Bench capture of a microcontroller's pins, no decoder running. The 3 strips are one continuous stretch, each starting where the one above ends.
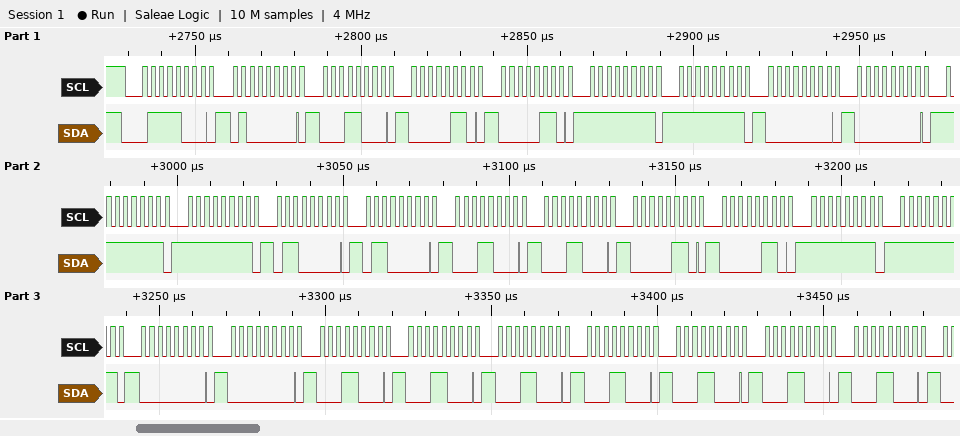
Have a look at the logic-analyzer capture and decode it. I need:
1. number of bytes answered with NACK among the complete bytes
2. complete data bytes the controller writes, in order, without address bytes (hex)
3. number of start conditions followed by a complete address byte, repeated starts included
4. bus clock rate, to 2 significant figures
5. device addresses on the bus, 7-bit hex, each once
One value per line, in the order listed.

0
40 18 06 06 FF FF 00 00 FF FF 60 60 18 18 06 06 FF FF 00 00 18 18 18 18 18 18 18
1
400 kHz
0x3C
